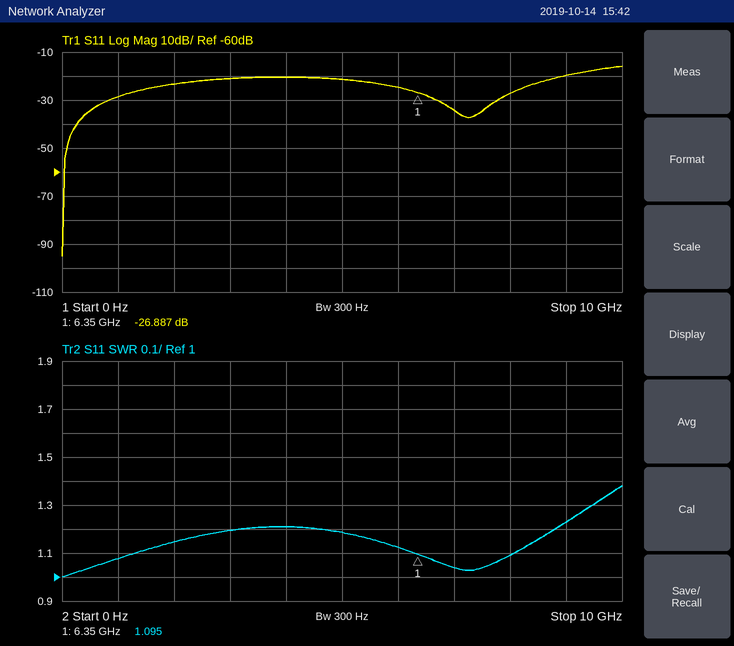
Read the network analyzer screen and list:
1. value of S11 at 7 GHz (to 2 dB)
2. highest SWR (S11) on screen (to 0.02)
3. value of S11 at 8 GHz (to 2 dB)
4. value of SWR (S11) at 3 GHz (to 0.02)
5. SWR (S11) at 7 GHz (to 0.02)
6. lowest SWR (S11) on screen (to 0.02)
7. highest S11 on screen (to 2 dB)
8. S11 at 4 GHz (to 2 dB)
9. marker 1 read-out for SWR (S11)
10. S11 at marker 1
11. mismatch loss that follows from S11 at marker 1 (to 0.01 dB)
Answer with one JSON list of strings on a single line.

["-34 dB", "1.38", "-28 dB", "1.20", "1.04", "1.00", "-16 dB", "-20 dB", "1.095", "-26.887 dB", "0.01 dB"]
